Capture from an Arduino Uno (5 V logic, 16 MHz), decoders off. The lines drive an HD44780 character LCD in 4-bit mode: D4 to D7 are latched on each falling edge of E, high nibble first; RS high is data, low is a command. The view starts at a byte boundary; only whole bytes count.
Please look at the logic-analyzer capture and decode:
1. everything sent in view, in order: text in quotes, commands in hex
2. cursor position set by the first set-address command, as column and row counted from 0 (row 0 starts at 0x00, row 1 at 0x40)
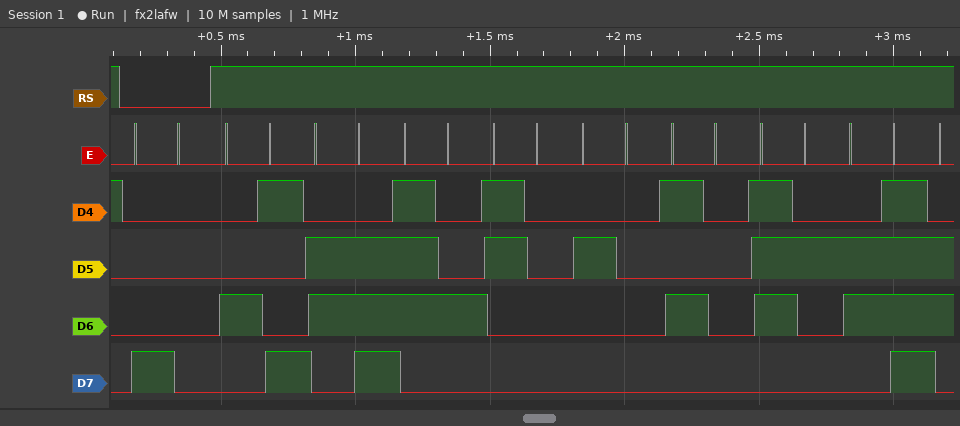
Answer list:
0x80 "Int0 Pro"
column 0, row 0
